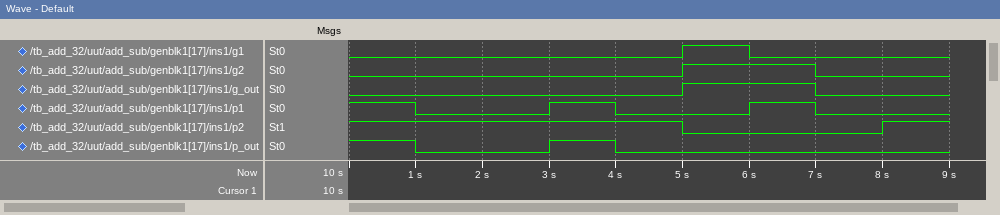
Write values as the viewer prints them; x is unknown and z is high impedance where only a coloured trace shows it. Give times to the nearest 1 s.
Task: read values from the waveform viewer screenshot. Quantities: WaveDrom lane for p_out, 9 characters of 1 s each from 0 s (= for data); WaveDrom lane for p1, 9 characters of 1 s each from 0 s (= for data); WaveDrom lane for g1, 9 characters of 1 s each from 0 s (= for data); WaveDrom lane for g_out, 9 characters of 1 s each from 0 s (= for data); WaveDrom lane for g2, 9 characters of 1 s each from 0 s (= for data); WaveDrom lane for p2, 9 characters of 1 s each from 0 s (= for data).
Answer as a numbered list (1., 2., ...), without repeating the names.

1. {name: 'p_out', wave: '10.10....'}
2. {name: 'p1', wave: '10.10.10.'}
3. {name: 'g1', wave: '0....10..'}
4. {name: 'g_out', wave: '0....1.0.'}
5. {name: 'g2', wave: '0....1.0.'}
6. {name: 'p2', wave: '1....0..1'}
